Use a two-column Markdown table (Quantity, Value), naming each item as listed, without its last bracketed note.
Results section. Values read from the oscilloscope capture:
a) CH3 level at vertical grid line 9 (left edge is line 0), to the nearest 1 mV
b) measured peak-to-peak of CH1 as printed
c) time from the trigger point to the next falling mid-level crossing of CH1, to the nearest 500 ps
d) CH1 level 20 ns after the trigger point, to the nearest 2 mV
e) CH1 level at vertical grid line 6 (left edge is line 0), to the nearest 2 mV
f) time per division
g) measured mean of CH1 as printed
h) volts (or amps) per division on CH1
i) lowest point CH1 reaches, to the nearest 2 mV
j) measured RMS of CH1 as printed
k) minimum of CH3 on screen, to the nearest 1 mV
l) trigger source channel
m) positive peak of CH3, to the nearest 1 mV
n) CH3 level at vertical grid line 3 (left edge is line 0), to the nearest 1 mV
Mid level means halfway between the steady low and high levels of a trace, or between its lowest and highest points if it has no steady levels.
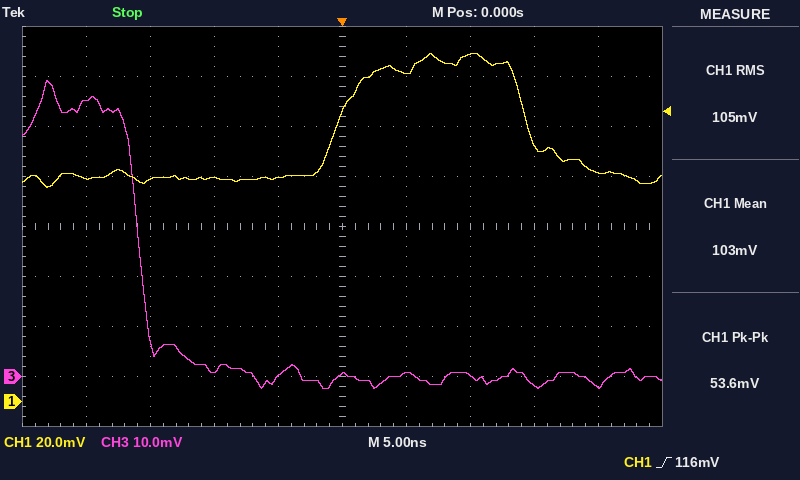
| Quantity | Value |
|---|---|
| CH3 level at vertical grid line 9 (left edge is line 0), to the nearest 1 mV | -2 mV |
| measured peak-to-peak of CH1 as printed | 53.6 mV |
| time from the trigger point to the next falling mid-level crossing of CH1, to the nearest 500 ps | 14.5 ns |
| CH1 level 20 ns after the trigger point, to the nearest 2 mV | 92 mV |
| CH1 level at vertical grid line 6 (left edge is line 0), to the nearest 2 mV | 132 mV |
| time per division | 5 ns |
| measured mean of CH1 as printed | 103 mV |
| volts (or amps) per division on CH1 | 20 mV |
| lowest point CH1 reaches, to the nearest 2 mV | 86 mV |
| measured RMS of CH1 as printed | 105 mV |
| minimum of CH3 on screen, to the nearest 1 mV | -2 mV |
| trigger source channel | CH1 |
| positive peak of CH3, to the nearest 1 mV | 59 mV |
| CH3 level at vertical grid line 3 (left edge is line 0), to the nearest 1 mV | 1 mV |
